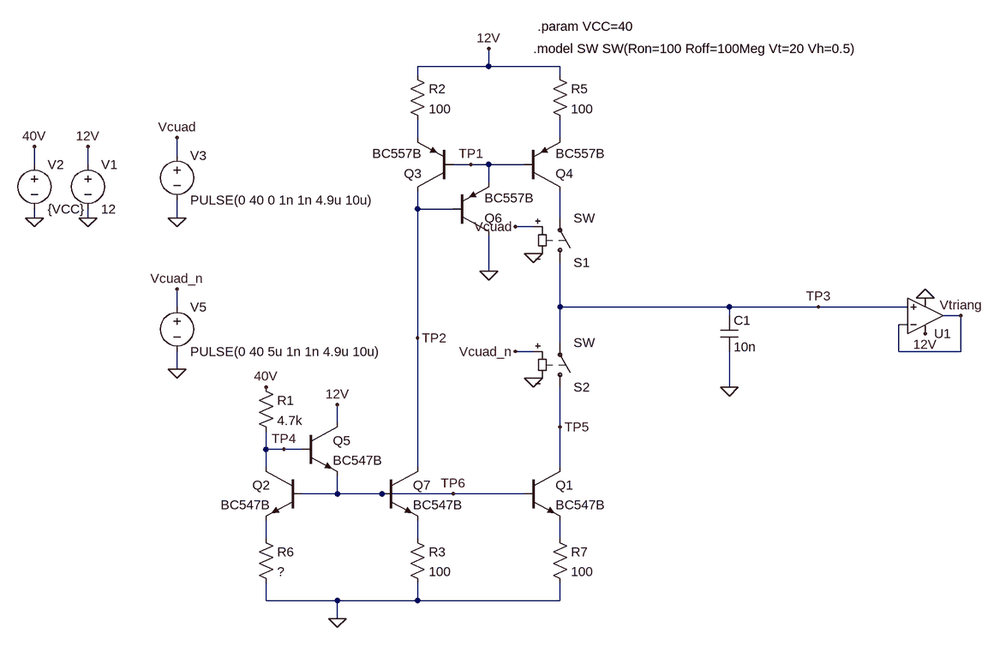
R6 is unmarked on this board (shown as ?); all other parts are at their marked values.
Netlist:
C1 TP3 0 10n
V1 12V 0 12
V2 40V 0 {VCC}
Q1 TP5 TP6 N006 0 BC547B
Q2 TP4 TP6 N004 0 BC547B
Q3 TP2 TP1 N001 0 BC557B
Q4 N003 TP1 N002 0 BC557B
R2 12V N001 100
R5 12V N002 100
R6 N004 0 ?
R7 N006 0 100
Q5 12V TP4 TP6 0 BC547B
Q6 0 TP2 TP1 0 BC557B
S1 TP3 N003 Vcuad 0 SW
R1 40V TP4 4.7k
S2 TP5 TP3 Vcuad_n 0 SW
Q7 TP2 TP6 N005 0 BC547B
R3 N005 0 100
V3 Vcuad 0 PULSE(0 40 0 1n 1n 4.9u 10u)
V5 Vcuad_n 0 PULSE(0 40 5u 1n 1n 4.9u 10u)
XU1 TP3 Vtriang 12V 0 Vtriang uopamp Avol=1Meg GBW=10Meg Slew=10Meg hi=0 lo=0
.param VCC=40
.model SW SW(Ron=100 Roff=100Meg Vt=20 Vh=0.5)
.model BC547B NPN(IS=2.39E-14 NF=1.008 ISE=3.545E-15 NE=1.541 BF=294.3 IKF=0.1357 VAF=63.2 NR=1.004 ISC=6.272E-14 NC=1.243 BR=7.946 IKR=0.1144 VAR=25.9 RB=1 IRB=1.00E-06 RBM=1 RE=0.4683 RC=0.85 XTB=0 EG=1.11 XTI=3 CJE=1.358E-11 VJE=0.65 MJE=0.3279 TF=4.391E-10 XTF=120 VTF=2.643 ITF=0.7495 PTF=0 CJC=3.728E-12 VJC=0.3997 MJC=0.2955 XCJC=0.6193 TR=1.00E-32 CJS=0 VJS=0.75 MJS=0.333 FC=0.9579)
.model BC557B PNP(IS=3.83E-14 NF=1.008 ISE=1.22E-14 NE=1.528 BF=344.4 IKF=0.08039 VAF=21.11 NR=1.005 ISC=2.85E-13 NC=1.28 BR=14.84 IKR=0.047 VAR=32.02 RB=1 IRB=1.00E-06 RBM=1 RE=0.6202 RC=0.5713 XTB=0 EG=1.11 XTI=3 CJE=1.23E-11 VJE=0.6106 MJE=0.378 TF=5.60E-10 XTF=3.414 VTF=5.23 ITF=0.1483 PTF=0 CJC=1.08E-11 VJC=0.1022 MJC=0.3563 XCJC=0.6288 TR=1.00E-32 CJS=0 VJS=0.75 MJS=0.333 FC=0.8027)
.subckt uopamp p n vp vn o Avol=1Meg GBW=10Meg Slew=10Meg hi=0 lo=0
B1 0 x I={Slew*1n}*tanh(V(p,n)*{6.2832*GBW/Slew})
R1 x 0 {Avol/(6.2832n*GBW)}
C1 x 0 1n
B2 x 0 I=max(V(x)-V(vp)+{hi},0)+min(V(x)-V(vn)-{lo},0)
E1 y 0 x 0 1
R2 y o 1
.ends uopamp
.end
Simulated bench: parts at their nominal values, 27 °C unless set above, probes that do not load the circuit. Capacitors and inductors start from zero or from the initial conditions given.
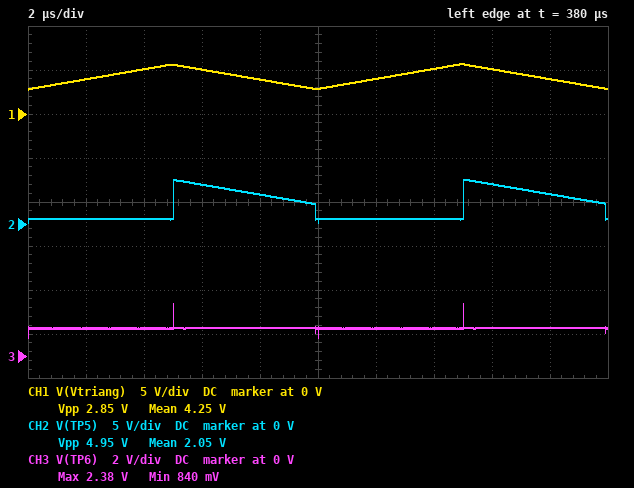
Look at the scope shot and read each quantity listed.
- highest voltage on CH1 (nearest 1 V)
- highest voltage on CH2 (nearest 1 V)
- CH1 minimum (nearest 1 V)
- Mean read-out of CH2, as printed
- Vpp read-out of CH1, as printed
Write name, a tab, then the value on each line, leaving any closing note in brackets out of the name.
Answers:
highest voltage on CH1	6 V
highest voltage on CH2	5 V
CH1 minimum	3 V
Mean read-out of CH2, as printed	2.05 V
Vpp read-out of CH1, as printed	2.85 V
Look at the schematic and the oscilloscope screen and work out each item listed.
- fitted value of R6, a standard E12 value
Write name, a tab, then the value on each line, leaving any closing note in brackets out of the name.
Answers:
fitted value of R6, a standard E12 value	68 Ω
